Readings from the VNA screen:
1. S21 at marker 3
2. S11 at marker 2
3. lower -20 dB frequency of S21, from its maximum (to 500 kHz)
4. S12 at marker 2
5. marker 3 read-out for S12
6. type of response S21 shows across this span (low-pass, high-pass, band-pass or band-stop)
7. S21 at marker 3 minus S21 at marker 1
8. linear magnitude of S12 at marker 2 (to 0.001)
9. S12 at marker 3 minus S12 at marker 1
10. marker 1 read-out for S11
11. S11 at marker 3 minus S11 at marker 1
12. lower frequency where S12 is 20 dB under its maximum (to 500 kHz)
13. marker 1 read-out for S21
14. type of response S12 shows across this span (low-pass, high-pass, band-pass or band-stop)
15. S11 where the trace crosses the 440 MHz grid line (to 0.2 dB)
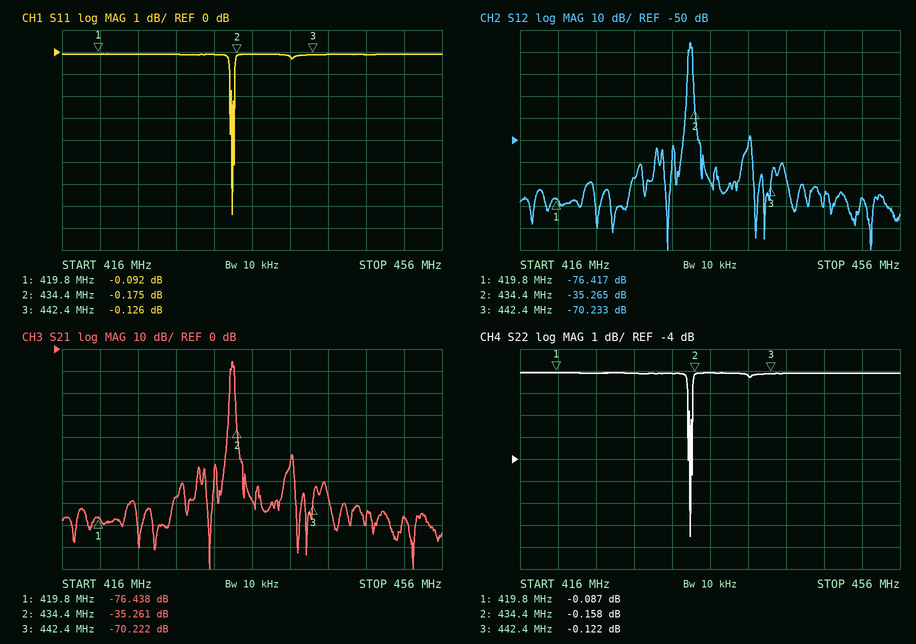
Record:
-70.222 dB
-0.175 dB
433.5 MHz
-35.265 dB
-70.233 dB
band-pass
6.216 dB
0.017
6.184 dB
-0.092 dB
-0.034 dB
433.5 MHz
-76.438 dB
band-pass
-0.2 dB
